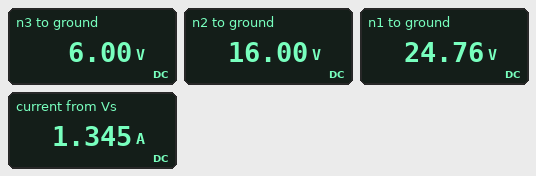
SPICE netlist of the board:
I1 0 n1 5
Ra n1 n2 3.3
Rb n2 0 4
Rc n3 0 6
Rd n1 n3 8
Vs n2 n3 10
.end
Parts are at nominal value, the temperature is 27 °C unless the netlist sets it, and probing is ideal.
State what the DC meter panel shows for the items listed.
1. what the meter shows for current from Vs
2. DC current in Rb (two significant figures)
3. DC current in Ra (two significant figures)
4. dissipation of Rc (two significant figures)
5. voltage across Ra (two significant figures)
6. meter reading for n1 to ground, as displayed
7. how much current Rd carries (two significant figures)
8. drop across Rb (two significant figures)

1.345 A
4.0 A
2.7 A
6.0 W
8.8 V
24.76 V
2.3 A
16 V
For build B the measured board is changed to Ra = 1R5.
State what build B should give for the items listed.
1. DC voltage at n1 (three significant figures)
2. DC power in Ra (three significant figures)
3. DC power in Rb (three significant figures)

20.7 V
15.0 W
64.0 W
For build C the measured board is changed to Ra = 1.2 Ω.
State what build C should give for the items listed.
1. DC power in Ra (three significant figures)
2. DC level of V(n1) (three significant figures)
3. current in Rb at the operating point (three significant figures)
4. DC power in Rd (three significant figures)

12.8 W
19.9 V
4.00 A
24.2 W
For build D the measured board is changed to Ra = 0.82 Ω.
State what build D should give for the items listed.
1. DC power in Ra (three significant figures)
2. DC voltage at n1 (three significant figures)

9.49 W
18.8 V
